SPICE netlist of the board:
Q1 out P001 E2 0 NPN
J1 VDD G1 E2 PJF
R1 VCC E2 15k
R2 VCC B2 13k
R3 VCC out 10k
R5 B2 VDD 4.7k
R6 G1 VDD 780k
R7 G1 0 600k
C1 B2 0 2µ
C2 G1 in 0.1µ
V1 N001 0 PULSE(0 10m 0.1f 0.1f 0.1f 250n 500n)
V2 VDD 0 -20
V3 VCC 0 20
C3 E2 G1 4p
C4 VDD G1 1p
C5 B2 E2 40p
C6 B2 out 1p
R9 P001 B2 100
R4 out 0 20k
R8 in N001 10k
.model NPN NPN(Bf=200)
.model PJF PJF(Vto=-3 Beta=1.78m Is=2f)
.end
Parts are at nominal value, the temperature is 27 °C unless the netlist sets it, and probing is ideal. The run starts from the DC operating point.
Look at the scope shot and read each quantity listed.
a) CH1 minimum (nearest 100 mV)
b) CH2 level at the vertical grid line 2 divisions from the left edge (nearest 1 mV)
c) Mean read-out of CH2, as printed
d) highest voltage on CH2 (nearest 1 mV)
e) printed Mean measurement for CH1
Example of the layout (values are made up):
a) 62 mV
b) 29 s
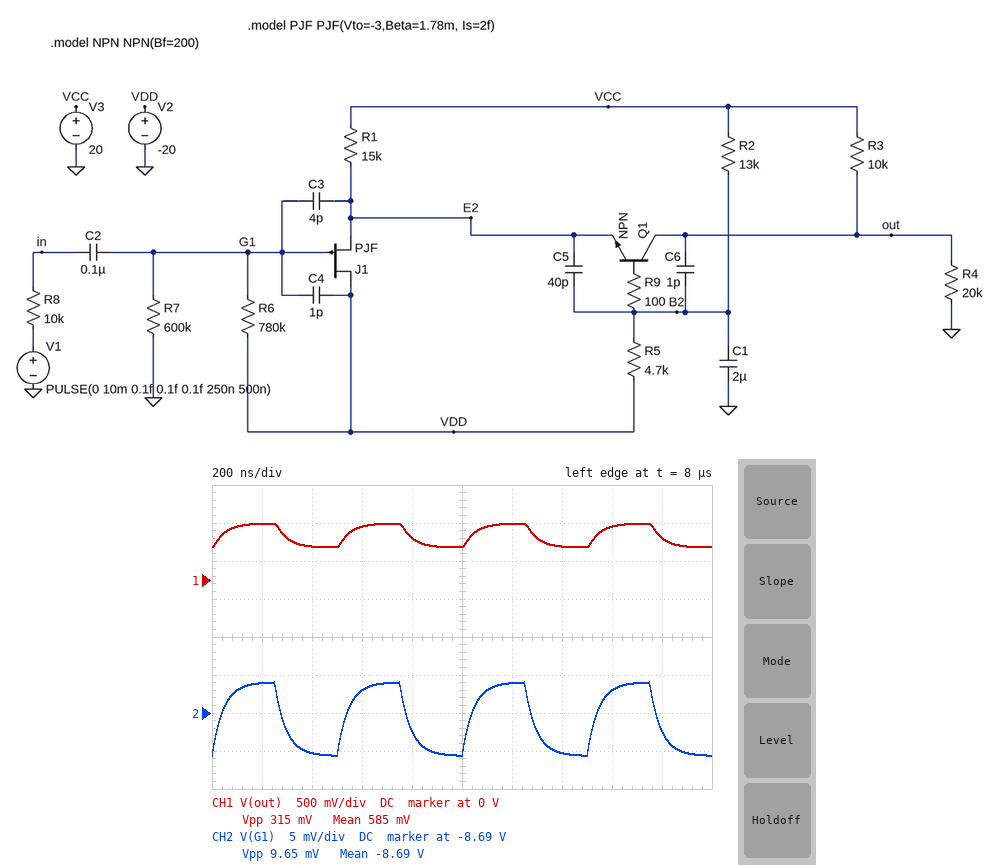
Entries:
a) 400 mV
b) -8.695 V
c) -8.69 V
d) -8.686 V
e) 585 mV
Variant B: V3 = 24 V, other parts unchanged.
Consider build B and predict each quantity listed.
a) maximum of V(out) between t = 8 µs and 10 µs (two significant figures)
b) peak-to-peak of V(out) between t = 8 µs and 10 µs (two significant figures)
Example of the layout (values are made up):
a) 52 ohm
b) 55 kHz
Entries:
a) -9.7 V
b) 9.6 mV
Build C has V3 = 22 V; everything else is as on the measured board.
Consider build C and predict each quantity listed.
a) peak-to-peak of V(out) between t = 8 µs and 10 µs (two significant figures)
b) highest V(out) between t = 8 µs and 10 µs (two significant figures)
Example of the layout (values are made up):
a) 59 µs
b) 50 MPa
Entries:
a) 36 mV
b) -9.7 V
